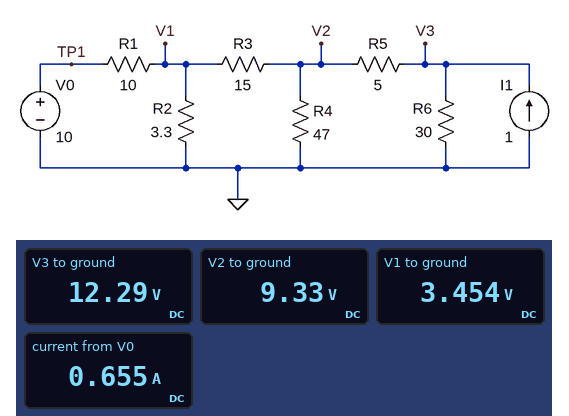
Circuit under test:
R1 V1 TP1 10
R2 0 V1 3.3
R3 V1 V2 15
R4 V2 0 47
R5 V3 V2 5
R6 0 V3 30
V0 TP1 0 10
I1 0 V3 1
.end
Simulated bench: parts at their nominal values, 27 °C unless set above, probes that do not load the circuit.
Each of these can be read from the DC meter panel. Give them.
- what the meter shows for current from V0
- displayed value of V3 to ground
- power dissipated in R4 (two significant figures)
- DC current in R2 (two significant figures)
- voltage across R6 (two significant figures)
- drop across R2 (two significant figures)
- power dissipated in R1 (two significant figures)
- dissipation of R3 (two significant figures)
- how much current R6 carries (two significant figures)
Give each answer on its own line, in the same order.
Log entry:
0.655 A
12.29 V
1.9 W
1.0 A
12 V
3.5 V
4.3 W
2.3 W
410 mA
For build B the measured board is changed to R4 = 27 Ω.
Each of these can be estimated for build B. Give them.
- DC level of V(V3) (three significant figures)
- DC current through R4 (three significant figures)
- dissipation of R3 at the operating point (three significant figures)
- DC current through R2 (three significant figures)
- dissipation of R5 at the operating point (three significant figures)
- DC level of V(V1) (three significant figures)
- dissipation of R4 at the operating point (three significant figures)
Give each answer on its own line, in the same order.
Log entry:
11.3 V
301 mA
1.57 W
995 mA
1.95 W
3.28 V
2.45 W
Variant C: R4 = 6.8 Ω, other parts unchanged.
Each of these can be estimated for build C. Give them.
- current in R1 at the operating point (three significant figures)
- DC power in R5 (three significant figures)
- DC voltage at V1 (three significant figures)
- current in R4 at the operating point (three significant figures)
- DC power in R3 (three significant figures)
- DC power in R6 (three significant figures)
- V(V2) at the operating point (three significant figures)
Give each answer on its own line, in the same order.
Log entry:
726 mA
2.70 W
2.74 V
631 mA
161 mW
2.11 W
4.29 V
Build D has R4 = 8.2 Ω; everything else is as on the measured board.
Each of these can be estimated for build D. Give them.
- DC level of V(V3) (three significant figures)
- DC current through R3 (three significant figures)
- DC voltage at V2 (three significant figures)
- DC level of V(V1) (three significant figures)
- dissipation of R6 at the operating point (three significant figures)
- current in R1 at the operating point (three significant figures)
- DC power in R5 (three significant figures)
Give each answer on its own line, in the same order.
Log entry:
8.41 V
133 mA
4.81 V
2.81 V
2.36 W
719 mA
2.59 W
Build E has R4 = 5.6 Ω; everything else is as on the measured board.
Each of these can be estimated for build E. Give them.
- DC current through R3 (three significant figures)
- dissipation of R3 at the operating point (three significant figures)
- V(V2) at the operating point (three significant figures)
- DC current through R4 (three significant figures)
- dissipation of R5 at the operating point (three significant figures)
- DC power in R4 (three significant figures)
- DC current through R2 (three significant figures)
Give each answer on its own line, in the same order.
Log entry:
74.3 mA
82.7 mW
3.78 V
675 mA
2.81 W
2.55 W
808 mA
